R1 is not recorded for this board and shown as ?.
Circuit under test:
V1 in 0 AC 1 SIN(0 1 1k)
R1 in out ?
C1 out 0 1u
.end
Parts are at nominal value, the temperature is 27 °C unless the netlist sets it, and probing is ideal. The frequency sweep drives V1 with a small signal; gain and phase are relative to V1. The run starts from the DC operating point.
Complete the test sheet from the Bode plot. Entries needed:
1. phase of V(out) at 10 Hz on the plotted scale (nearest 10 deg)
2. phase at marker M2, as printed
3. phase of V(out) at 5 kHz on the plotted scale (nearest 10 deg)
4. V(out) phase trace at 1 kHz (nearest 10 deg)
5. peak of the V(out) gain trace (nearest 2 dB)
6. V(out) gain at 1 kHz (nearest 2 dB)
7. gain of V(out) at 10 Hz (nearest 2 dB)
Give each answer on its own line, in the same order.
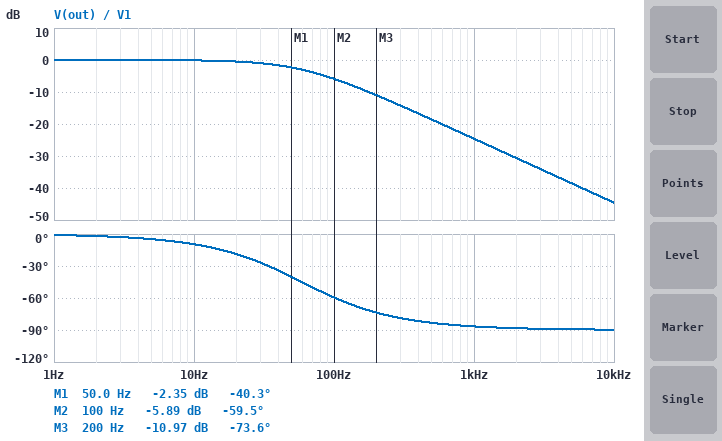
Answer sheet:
-10 deg
-59.5 deg
-90 deg
-90 deg
0 dB
-24 dB
0 dB
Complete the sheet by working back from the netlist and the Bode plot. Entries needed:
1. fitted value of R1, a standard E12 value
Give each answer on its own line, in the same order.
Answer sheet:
2.7 kΩ
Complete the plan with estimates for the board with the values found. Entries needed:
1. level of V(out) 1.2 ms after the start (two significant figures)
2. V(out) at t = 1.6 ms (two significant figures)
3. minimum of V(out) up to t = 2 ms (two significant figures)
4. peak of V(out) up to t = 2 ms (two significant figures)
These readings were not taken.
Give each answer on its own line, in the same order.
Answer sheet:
23 mV
78 mV
-31 mV
110 mV
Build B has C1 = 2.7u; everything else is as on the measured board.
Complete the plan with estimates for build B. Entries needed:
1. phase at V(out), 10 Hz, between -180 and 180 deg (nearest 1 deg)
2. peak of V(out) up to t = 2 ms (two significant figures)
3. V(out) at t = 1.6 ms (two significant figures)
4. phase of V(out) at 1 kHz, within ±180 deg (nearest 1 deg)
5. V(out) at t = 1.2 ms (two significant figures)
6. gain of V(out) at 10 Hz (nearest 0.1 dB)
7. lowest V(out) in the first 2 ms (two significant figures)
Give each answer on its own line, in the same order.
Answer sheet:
-25 deg
42 mV
35 mV
-89 deg
12 mV
-0.8 dB
-5.2 mV
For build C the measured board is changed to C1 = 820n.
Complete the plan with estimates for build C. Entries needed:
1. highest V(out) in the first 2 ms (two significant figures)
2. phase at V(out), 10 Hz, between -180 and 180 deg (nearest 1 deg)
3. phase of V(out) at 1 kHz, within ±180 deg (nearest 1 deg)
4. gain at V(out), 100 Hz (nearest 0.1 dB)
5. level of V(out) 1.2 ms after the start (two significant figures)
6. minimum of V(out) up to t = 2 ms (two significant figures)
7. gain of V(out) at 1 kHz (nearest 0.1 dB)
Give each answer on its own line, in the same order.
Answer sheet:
130 mV
-8 deg
-86 deg
-4.7 dB
24 mV
-43 mV
-22.9 dB
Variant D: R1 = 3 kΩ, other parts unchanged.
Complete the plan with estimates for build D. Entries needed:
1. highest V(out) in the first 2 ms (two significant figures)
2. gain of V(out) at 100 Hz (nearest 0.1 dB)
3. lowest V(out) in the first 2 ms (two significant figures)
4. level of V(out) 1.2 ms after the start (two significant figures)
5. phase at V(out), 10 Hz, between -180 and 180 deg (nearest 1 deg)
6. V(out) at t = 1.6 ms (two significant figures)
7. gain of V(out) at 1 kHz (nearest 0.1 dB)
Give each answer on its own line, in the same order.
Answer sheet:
98 mV
-6.6 dB
-26 mV
22 mV
-11 deg
72 mV
-25.5 dB
